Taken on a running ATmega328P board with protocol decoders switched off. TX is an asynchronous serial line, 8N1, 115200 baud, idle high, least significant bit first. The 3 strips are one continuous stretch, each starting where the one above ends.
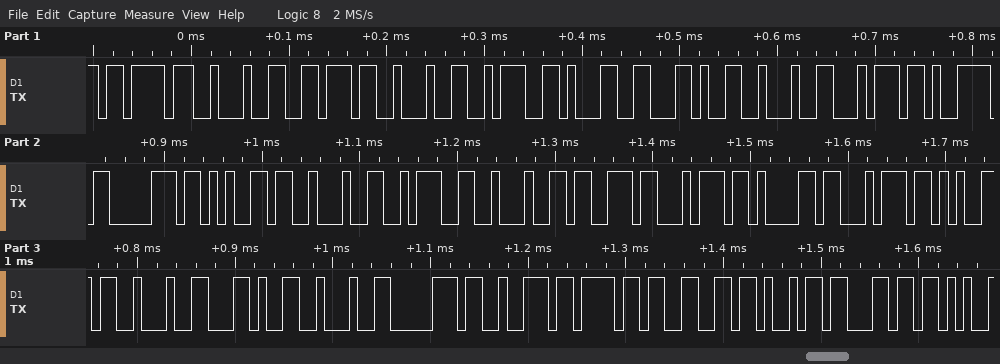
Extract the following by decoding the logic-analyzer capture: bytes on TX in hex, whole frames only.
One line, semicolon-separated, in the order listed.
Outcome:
7B 22 76 22 3A 31 2C 22 74 79 70 65 22 3A 22 73 74 61 74 65 22 2C 22 70 72 6F 66 69 6C
